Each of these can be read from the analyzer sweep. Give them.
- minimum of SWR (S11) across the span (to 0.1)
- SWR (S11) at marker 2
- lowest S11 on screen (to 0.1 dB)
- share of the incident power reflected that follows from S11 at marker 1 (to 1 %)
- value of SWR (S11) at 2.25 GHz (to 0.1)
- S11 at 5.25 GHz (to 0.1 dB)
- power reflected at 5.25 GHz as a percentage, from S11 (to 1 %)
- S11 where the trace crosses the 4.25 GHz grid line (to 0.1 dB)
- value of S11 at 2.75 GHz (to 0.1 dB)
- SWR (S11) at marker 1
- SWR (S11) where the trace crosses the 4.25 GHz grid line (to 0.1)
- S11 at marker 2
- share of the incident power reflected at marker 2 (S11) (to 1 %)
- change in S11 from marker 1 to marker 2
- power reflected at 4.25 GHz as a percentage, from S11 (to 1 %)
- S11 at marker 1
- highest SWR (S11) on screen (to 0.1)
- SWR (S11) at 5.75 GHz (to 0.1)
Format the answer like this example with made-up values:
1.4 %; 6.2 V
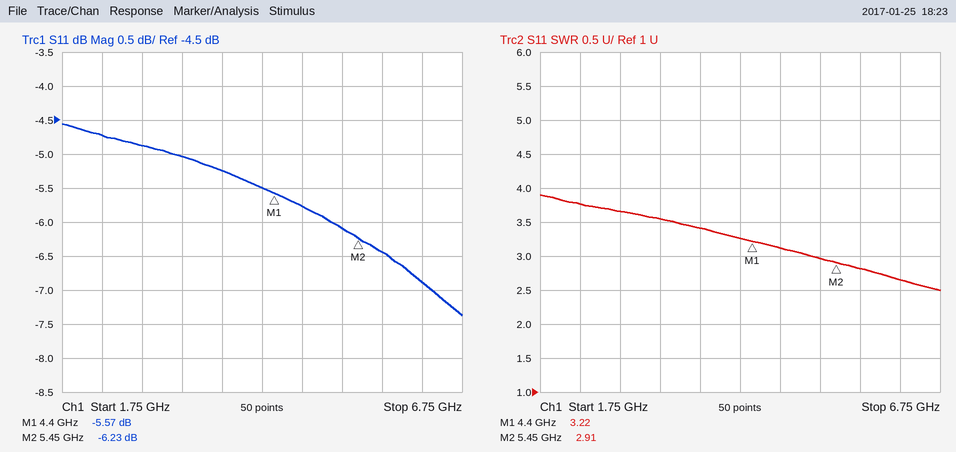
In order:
2.5; 2.91; -7.4 dB; 28 %; 3.8; -6.1 dB; 25 %; -5.5 dB; -4.9 dB; 3.22; 3.3; -6.23 dB; 24 %; -0.66 dB; 28 %; -5.57 dB; 3.9; 2.8
